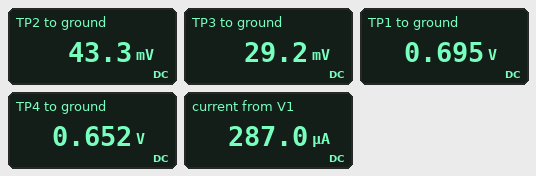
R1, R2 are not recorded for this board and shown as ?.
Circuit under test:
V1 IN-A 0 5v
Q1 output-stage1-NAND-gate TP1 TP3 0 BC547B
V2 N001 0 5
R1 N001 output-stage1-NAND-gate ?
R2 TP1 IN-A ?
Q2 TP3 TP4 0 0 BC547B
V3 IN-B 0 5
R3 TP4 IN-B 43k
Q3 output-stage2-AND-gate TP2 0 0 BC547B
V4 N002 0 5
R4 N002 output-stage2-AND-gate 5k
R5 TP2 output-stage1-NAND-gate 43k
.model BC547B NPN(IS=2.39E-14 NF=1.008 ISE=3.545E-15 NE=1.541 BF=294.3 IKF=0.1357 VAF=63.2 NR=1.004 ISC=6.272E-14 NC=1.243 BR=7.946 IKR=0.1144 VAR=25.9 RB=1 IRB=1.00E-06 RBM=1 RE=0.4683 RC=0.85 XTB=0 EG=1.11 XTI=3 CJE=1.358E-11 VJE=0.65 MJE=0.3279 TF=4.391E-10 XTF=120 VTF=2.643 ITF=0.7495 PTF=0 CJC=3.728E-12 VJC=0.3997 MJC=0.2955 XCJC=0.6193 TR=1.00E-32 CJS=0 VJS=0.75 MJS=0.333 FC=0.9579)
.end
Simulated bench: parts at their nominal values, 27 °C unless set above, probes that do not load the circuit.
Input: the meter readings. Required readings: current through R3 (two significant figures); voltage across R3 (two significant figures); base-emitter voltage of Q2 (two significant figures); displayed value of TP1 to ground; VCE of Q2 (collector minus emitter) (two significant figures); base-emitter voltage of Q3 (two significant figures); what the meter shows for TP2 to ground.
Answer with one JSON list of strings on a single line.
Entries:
["100 µA", "4.3 V", "650 mV", "0.695 V", "29 mV", "43 mV", "43.3 mV"]
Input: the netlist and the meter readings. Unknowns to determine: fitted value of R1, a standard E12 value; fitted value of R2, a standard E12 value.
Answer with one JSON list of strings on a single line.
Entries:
["8.2 kΩ", "15 kΩ"]
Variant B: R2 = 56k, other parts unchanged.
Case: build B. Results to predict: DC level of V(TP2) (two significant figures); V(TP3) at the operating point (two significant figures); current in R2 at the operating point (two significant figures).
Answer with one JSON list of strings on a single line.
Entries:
["52 mV", "25 mV", "77 µA"]
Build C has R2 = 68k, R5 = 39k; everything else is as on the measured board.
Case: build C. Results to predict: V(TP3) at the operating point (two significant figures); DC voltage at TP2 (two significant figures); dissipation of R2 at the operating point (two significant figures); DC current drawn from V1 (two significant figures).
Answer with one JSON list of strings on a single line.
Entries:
["25 mV", "55 mV", "280 µW", "64 µA"]
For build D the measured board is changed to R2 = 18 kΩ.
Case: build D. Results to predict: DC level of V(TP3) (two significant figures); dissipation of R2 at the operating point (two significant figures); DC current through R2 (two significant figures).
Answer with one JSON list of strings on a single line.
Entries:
["28 mV", "1.0 mW", "240 µA"]
